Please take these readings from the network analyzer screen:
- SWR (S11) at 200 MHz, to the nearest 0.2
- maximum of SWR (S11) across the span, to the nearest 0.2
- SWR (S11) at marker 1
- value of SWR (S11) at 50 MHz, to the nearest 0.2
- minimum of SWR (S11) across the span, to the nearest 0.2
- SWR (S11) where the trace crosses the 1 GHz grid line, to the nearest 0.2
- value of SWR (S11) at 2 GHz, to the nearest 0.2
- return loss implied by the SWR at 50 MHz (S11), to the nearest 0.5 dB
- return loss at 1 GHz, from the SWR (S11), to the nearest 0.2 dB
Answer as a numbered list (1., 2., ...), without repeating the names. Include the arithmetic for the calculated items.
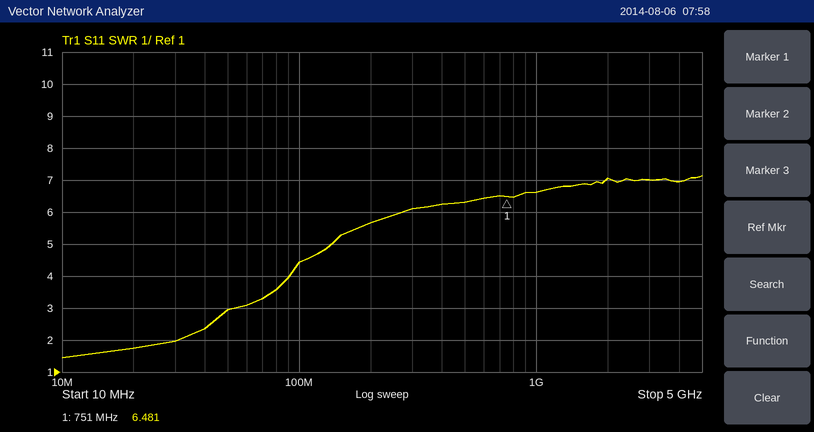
1. 5.6
2. 7.2
3. 6.481
4. 3.0
5. 1.4
6. 6.6
7. 7.0
8. −20 log10((3 − 1)/(3 + 1)) ≈ 6.0 dB
9. −20 log10((6.6 − 1)/(6.6 + 1)) ≈ 2.6 dB
